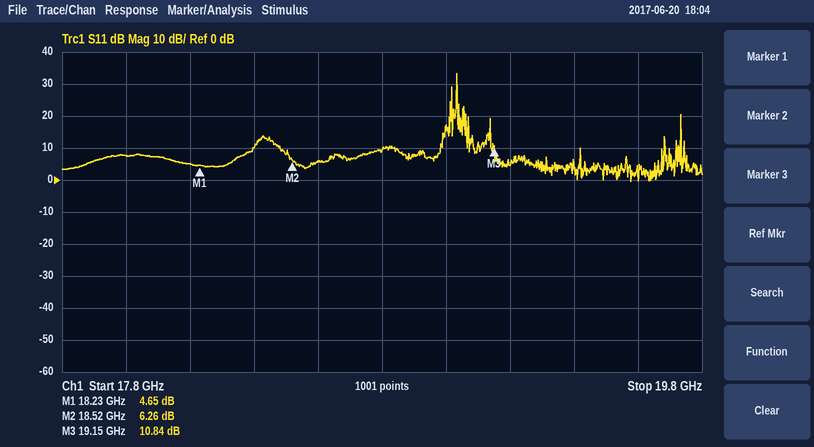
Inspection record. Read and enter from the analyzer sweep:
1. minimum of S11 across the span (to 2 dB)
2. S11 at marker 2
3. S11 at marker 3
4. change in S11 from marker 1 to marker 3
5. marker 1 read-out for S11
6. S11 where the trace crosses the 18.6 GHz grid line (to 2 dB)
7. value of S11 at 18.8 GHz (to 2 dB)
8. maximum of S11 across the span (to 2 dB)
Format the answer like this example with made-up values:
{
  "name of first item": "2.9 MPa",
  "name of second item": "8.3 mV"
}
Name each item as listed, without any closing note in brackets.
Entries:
{
  "minimum of S11 across the span": "0 dB",
  "S11 at marker 2": "6.26 dB",
  "S11 at marker 3": "10.84 dB",
  "change in S11 from marker 1 to marker 3": "6.19 dB",
  "marker 1 read-out for S11": "4.65 dB",
  "S11 where the trace crosses the 18.6 GHz grid line": "6 dB",
  "value of S11 at 18.8 GHz": "10 dB",
  "maximum of S11 across the span": "34 dB"
}
